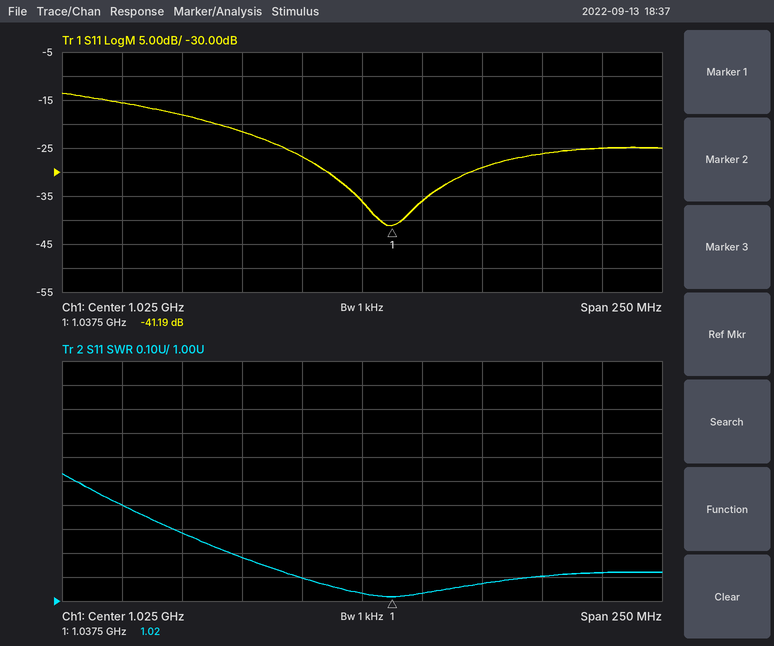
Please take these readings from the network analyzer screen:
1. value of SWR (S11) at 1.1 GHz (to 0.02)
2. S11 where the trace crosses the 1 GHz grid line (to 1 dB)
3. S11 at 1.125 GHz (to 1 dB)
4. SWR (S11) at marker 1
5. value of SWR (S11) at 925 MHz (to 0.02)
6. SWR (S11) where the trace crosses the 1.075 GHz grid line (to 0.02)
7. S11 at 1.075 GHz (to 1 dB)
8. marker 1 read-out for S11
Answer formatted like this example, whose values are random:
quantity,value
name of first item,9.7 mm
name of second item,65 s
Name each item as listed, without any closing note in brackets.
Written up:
quantity,value
value of SWR (S11) at 1.1 GHz,1.10
S11 where the trace crosses the 1 GHz grid line,-27 dB
S11 at 1.125 GHz,-25 dB
SWR (S11) at marker 1,1.02
value of SWR (S11) at 925 MHz,1.40
SWR (S11) where the trace crosses the 1.075 GHz grid line,1.08
S11 at 1.075 GHz,-29 dB
marker 1 read-out for S11,-41.19 dB
